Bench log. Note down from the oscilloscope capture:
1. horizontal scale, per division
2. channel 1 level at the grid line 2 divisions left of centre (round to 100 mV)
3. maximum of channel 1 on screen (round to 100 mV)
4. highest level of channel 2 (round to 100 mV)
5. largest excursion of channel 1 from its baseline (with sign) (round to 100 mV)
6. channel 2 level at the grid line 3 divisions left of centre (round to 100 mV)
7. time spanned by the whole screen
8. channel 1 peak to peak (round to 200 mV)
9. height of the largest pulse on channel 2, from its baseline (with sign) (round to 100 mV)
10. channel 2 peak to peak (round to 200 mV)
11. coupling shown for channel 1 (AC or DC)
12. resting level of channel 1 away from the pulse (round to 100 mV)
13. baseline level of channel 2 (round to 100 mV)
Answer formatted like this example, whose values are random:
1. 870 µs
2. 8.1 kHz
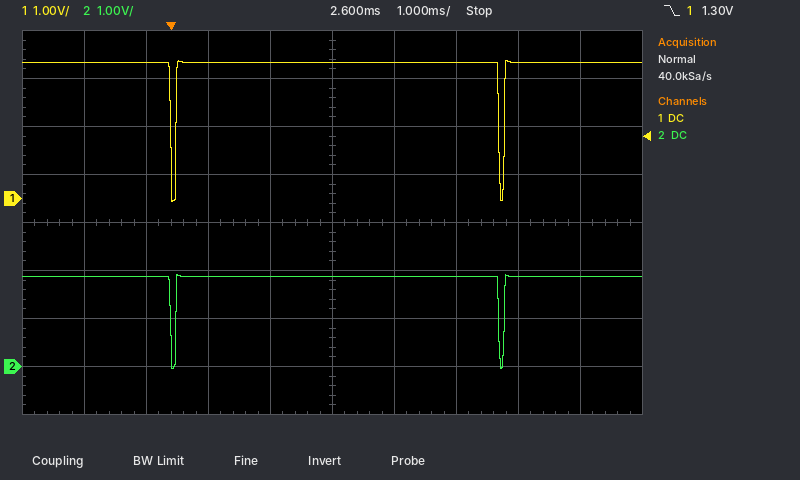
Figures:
1. 1 ms
2. 2.8 V
3. 2.9 V
4. 1.9 V
5. -2.9 V
6. 1.9 V
7. 10 ms
8. 3.0 V
9. -1.9 V
10. 2.0 V
11. DC
12. 2.8 V
13. 1.9 V
